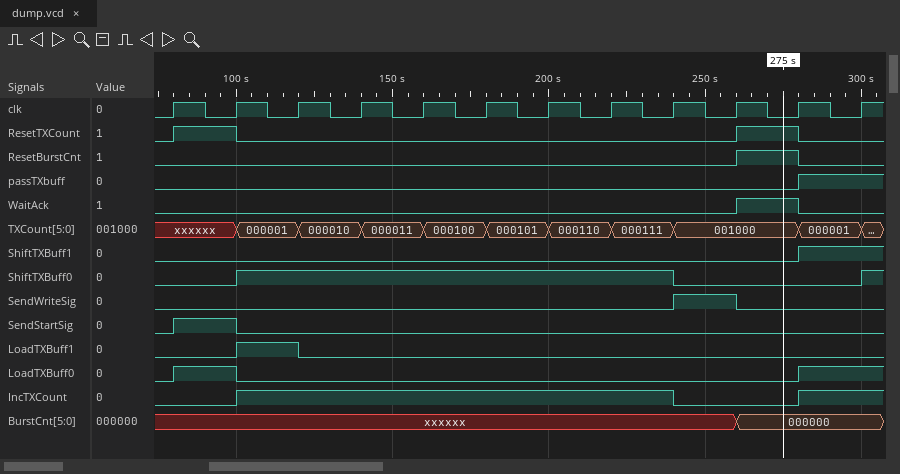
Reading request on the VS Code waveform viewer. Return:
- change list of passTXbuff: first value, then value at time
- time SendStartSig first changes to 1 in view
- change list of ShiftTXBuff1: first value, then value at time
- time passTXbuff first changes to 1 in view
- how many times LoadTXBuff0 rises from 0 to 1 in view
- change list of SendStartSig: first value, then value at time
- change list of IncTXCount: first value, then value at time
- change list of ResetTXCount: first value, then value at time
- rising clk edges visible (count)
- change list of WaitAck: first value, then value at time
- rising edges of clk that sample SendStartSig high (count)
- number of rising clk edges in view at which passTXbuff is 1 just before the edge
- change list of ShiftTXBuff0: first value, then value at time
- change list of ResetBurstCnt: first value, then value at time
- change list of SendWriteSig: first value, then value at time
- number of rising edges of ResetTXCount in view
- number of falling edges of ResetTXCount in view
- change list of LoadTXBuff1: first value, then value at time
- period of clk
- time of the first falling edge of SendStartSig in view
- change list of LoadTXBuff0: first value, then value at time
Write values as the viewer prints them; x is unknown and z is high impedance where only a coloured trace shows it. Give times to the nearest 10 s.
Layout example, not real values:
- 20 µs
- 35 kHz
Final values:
- 0, 1 at 280 s
- 80 s
- 0, 1 at 280 s
- 280 s
- 2
- 0, 1 at 80 s, 0 at 100 s
- 0, 1 at 100 s, 0 at 240 s, 1 at 280 s
- 0, 1 at 80 s, 0 at 100 s, 1 at 260 s, 0 at 280 s
- 12
- 0, 1 at 260 s, 0 at 280 s
- 1
- 1
- 0, 1 at 100 s, 0 at 240 s, 1 at 300 s
- 0, 1 at 260 s, 0 at 280 s
- 0, 1 at 240 s, 0 at 260 s
- 2
- 2
- 0, 1 at 100 s, 0 at 120 s
- 20 s
- 100 s
- 0, 1 at 80 s, 0 at 100 s, 1 at 280 s
